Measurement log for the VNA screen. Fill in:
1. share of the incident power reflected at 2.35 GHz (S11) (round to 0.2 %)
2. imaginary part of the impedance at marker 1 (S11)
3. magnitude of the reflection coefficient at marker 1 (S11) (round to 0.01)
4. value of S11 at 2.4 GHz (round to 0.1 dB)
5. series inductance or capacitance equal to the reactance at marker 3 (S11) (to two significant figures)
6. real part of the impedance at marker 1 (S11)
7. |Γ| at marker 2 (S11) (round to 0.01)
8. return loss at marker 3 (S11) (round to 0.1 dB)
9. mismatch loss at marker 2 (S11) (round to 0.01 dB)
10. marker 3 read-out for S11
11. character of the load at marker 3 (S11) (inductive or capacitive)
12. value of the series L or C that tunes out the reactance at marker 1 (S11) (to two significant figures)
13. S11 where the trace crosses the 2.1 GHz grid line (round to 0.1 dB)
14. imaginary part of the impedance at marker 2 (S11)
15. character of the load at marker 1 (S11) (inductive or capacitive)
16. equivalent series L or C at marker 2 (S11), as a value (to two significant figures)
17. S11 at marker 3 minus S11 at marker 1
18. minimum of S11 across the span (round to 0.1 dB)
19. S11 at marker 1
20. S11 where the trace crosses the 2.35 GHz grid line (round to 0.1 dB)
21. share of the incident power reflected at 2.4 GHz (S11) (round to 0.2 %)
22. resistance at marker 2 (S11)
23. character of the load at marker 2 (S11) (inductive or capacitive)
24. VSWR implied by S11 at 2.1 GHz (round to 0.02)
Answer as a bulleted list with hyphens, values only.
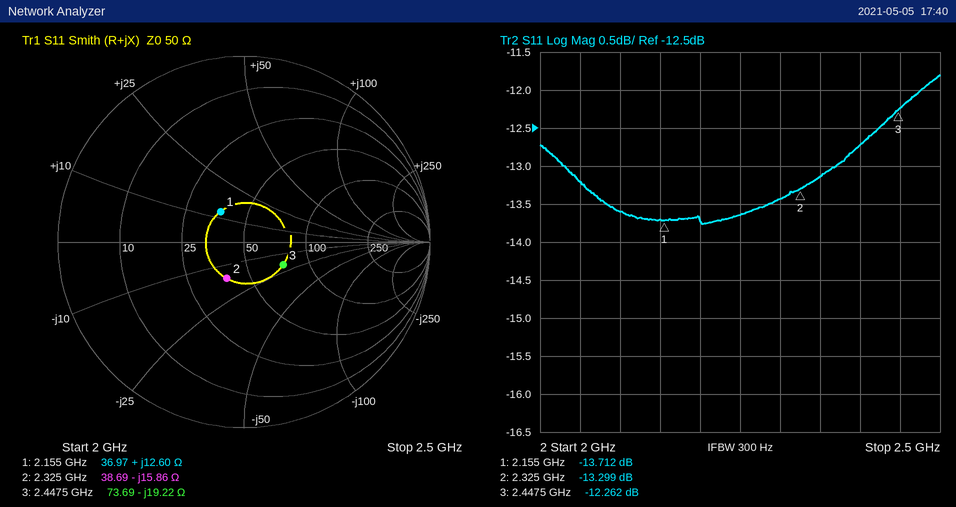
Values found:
- 4.8 %
- +12.60 Ω
- 0.21
- -12.7 dB
- 3.4 pF
- 36.97 Ω
- 0.22
- 12.3 dB
- 0.21 dB
- -12.262 dB
- capacitive
- 5.9 pF
- -13.6 dB
- -15.86 Ω
- inductive
- 4.3 pF
- 1.450 dB
- -13.8 dB
- -13.712 dB
- -13.1 dB
- 5.4 %
- 38.69 Ω
- capacitive
- 1.52
